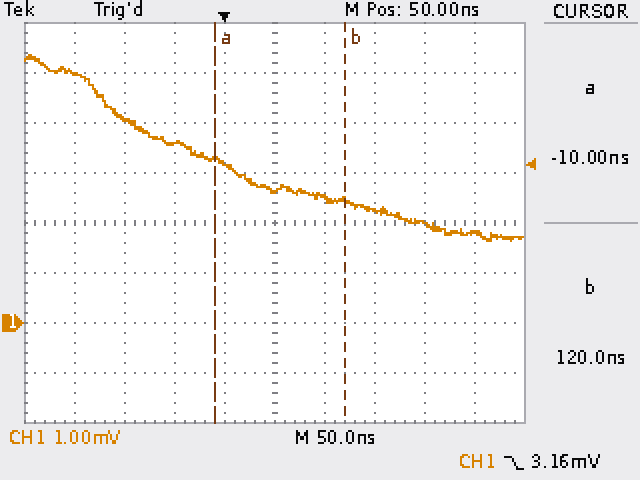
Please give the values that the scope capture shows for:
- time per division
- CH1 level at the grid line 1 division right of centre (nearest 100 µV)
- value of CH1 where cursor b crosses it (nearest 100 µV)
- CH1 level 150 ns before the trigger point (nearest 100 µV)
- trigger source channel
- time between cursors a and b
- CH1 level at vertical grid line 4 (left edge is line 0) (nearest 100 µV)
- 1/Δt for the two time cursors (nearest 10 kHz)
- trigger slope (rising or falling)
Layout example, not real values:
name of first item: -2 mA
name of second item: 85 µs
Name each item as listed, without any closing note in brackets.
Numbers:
time per division: 50 ns
CH1 level at the grid line 1 division right of centre: 2.5 mV
value of CH1 where cursor b crosses it: 2.4 mV
CH1 level 150 ns before the trigger point: 5.0 mV
trigger source channel: CH1
time between cursors a and b: 130 ns
CH1 level at vertical grid line 4 (left edge is line 0): 3.2 mV
1/Δt for the two time cursors: 7.69 MHz
trigger slope: falling
